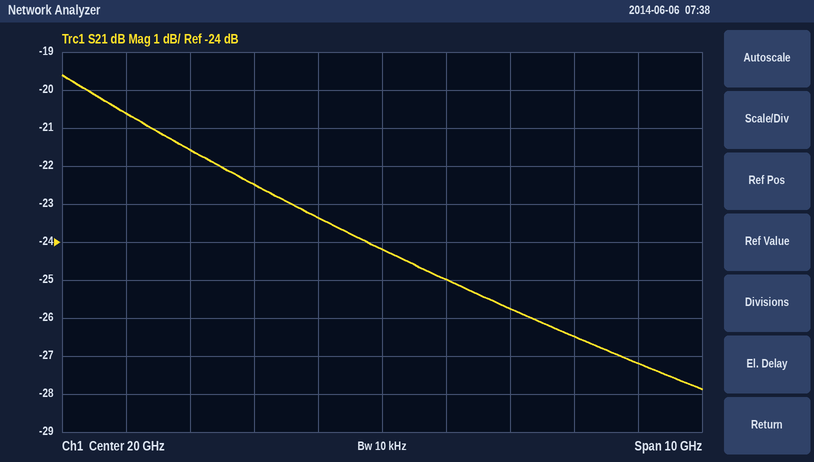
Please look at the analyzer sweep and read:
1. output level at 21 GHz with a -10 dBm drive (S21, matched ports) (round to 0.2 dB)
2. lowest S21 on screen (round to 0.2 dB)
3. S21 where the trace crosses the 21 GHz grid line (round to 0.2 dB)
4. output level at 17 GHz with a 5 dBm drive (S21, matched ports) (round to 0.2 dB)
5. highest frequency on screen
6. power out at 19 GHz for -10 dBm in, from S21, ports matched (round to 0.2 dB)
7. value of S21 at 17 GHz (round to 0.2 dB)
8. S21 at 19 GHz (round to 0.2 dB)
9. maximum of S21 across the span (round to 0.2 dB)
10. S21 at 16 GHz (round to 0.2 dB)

-35.0 dBm
-27.8 dB
-25.0 dB
-16.6 dBm
25 GHz
-33.4 dBm
-21.6 dB
-23.4 dB
-19.6 dB
-20.6 dB
